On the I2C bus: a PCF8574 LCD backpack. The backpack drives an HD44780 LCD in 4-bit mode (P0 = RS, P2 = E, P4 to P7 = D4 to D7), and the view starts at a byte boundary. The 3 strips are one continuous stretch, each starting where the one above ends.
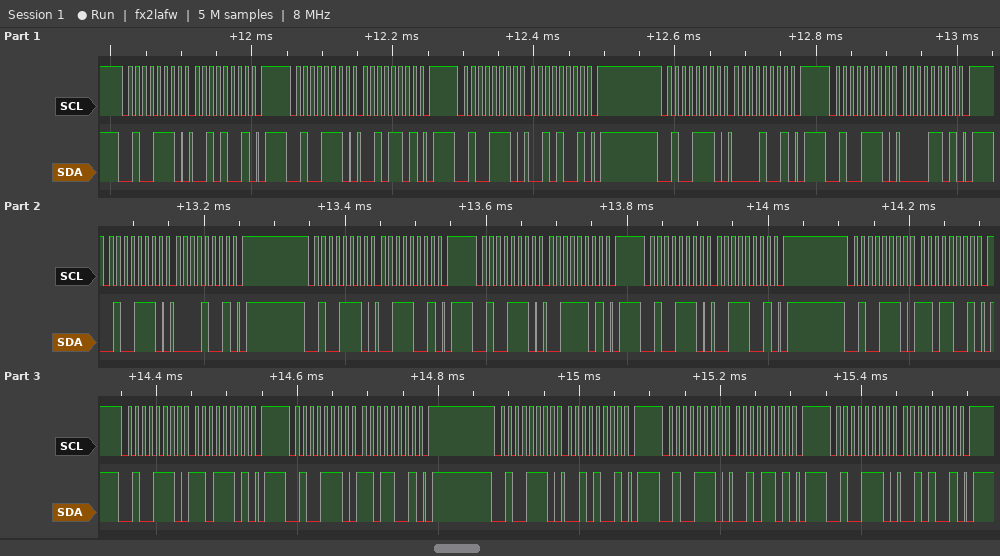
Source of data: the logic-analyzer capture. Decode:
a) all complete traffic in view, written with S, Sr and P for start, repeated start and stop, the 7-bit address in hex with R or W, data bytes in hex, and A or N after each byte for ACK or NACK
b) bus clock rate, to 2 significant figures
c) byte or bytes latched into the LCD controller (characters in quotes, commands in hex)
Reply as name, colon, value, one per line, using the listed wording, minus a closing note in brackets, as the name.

all complete traffic in view, written with S, Sr and P for start, repeated start and stop, the 7-bit address in hex with R or W, data bytes in hex, and A or N after each byte for ACK or NACK: S 27W A 29 A P S 27W A 2D A P S 27W A 29 A P S 27W A 09 A P S 27W A 0D A P S 27W A 09 A P S 27W A 39 A P S 27W A 3D A P S 27W A 39 A P S 27W A D9 A P S 27W A DD A P S 27W A D9 A P S 27W A 29 A P S 27W A 2D A P S 27W A 29 A P
bus clock rate, to 2 significant figures: 100 kHz
byte or bytes latched into the LCD controller: ' ' '='
